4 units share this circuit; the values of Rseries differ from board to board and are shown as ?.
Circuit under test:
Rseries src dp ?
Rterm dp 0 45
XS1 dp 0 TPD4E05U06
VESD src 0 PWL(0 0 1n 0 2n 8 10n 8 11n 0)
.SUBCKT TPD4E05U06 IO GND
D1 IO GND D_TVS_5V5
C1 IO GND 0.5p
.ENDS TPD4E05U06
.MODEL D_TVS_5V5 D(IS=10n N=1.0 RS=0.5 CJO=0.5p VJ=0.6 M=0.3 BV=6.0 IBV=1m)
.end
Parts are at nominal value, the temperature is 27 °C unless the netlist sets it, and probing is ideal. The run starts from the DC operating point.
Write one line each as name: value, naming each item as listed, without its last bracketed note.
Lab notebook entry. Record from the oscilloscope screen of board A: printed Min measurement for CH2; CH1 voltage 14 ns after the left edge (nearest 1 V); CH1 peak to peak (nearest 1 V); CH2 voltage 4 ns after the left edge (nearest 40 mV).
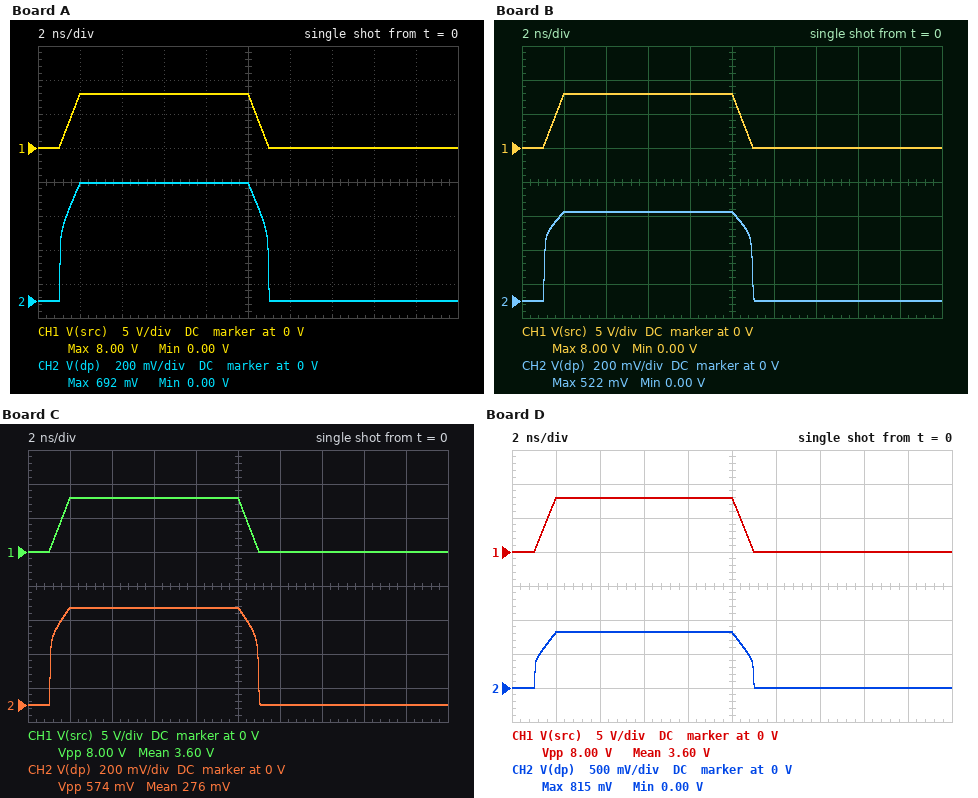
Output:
printed Min measurement for CH2: 0.00 V
CH1 voltage 14 ns after the left edge: 0 V
CH1 peak to peak: 8 V
CH2 voltage 4 ns after the left edge: 680 mV
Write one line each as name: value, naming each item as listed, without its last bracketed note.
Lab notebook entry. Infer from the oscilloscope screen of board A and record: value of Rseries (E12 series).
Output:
value of Rseries: 15 Ω
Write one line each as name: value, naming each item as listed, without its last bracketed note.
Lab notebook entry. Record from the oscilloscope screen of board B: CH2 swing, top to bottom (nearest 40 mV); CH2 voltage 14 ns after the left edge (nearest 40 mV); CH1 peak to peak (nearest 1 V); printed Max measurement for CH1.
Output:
CH2 swing, top to bottom: 520 mV
CH2 voltage 14 ns after the left edge: 0 V
CH1 peak to peak: 8 V
printed Max measurement for CH1: 8.00 V
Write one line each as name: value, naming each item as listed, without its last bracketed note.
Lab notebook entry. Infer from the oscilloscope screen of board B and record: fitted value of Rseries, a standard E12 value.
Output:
fitted value of Rseries, a standard E12 value: 39 Ω
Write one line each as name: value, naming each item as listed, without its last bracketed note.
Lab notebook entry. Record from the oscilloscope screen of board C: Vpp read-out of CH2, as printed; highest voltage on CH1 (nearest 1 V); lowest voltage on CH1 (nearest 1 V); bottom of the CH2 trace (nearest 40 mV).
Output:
Vpp read-out of CH2, as printed: 574 mV
highest voltage on CH1: 8 V
lowest voltage on CH1: 0 V
bottom of the CH2 trace: 0 V
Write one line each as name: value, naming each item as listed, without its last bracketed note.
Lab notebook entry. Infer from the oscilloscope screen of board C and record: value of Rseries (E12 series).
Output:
value of Rseries: 27 Ω
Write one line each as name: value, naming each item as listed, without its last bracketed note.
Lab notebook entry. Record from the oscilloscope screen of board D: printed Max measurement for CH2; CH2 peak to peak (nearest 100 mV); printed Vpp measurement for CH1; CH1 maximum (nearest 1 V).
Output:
printed Max measurement for CH2: 815 mV
CH2 peak to peak: 800 mV
printed Vpp measurement for CH1: 8.00 V
CH1 maximum: 8 V
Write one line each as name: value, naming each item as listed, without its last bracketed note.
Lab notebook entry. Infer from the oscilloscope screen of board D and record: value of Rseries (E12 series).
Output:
value of Rseries: 10 Ω
